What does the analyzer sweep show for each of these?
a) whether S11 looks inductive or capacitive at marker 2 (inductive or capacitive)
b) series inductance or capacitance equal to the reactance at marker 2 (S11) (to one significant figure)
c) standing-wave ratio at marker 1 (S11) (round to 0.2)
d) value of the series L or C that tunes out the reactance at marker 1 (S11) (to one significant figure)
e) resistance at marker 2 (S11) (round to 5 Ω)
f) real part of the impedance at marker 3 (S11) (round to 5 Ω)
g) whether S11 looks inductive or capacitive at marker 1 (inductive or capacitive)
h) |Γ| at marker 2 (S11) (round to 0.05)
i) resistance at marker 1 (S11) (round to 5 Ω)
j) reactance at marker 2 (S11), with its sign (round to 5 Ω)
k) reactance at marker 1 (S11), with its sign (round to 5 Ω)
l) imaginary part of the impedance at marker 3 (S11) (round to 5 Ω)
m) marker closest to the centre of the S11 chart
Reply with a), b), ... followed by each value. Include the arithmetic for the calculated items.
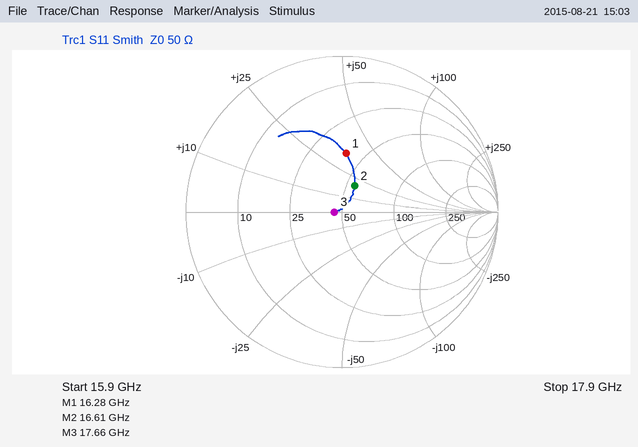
a) inductive
b) L = 20 Ω/(2π × 16.61 GHz) ≈ 192 pH, so 200 pH to one significant figure
c) 2.2
d) C = 1/(2π × 16.28 GHz × 35 Ω) ≈ 279 fF, so 300 fF to one significant figure
e) 55 Ω
f) 45 Ω
g) inductive
h) 0.20
i) 40 Ω
j) +20 Ω
k) +35 Ω
l) 0 Ω
m) marker 3
